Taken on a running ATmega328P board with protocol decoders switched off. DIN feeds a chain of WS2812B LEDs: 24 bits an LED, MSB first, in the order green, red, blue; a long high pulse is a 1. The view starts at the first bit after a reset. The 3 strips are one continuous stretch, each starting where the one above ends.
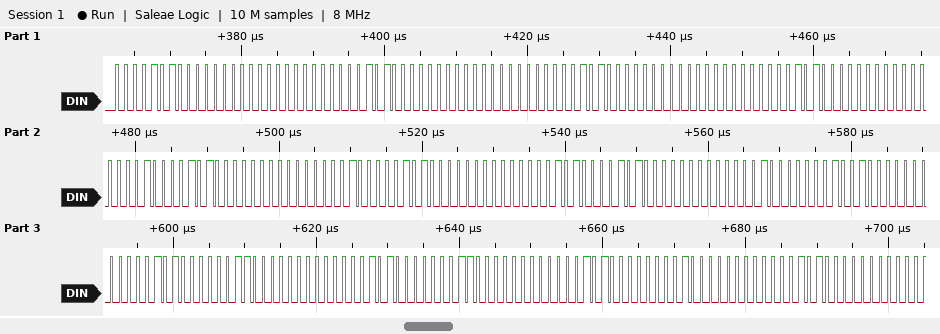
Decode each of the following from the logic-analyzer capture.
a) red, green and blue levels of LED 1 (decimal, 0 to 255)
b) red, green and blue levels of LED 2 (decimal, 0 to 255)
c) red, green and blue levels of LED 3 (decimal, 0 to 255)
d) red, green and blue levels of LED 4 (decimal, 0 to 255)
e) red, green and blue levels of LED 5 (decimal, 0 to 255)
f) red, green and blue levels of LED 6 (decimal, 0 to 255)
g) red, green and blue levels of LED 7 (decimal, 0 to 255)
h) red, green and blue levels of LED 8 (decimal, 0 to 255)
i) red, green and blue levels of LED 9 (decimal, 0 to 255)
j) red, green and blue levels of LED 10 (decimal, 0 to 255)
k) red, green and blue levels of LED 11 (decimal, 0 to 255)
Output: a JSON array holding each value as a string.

["0, 10, 0", "0, 10, 0", "0, 10, 0", "0, 10, 1", "0, 10, 2", "0, 10, 5", "0, 10, 8", "0, 9, 10", "0, 6, 10", "0, 3, 10", "0, 1, 10"]
